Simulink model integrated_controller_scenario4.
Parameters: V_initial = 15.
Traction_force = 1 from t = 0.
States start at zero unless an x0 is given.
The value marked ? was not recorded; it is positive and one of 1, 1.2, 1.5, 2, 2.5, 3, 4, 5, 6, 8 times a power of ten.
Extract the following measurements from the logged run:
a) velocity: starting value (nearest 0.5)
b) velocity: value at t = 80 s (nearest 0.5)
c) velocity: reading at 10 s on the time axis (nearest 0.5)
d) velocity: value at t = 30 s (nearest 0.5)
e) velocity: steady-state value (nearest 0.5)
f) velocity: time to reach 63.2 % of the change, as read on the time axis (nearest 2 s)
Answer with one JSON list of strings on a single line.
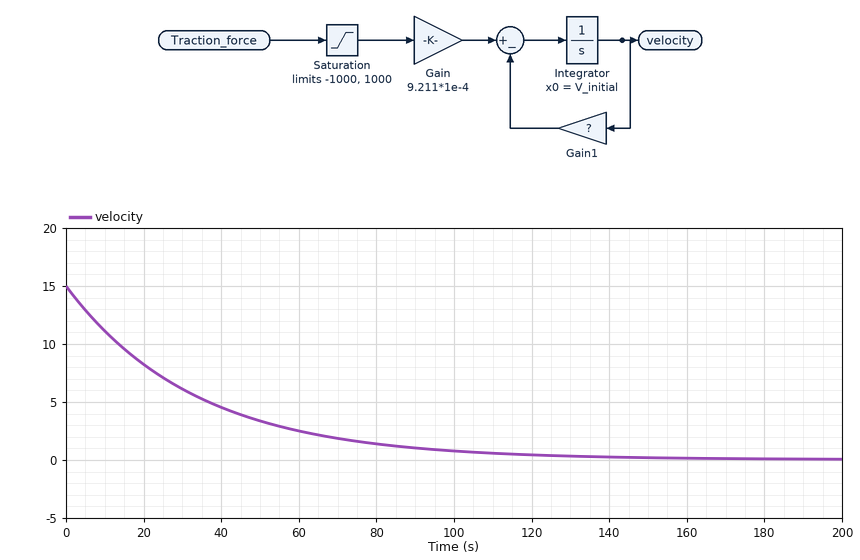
["15.0", "1.5", "11.0", "6.0", "0.0", "34 s"]
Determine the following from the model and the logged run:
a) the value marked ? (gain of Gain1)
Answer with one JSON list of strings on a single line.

["0.03"]
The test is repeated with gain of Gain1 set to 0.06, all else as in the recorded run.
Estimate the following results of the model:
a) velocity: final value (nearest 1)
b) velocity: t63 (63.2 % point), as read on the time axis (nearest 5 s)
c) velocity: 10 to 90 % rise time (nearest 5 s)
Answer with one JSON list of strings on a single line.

["0", "15 s", "35 s"]
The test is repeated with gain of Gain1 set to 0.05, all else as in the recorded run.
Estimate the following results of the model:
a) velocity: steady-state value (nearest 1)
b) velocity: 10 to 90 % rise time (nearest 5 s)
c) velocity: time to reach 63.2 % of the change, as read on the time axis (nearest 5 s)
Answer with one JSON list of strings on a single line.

["0", "45 s", "20 s"]
